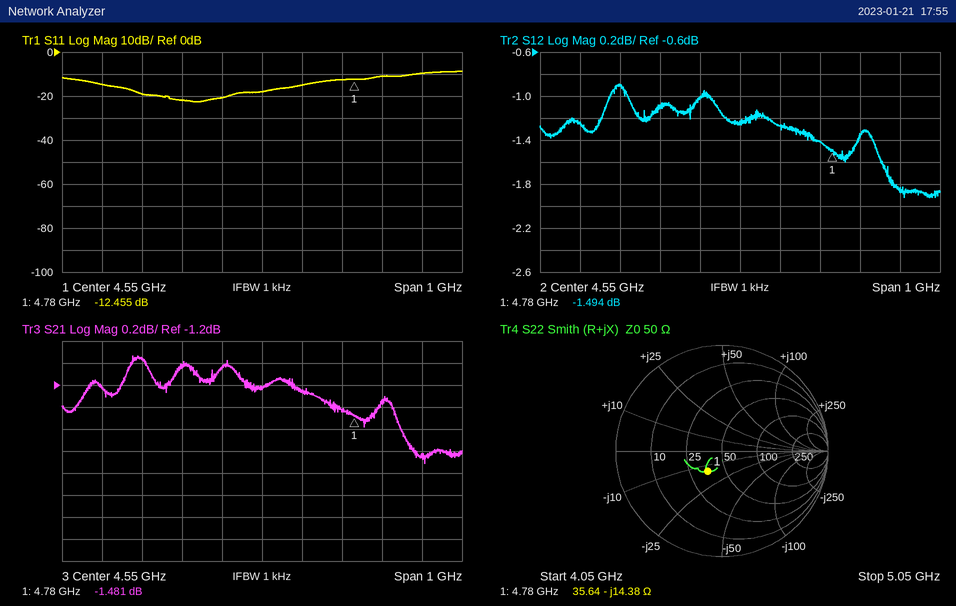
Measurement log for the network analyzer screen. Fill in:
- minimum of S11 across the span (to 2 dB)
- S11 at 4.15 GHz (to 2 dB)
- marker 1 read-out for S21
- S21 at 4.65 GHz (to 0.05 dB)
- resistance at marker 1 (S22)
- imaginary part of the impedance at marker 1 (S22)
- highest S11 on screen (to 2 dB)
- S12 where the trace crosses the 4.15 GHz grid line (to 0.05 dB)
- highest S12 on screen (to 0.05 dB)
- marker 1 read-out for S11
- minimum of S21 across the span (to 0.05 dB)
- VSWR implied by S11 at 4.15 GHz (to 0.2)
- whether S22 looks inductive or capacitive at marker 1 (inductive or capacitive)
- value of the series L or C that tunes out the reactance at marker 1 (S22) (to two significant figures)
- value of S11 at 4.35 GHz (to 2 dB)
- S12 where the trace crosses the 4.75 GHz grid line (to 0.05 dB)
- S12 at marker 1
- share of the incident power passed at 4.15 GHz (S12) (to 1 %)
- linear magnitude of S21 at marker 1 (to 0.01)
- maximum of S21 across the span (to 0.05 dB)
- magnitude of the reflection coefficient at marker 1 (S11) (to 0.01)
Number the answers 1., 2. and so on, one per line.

1. -22 dB
2. -14 dB
3. -1.481 dB
4. -1.25 dB
5. 35.64 Ω
6. -14.38 Ω
7. -8 dB
8. -1.25 dB
9. -0.90 dB
10. -12.455 dB
11. -1.90 dB
12. 1.4
13. capacitive
14. 480 pH
15. -22 dB
16. -1.40 dB
17. -1.494 dB
18. 75 %
19. 0.84
20. -0.95 dB
21. 0.24
